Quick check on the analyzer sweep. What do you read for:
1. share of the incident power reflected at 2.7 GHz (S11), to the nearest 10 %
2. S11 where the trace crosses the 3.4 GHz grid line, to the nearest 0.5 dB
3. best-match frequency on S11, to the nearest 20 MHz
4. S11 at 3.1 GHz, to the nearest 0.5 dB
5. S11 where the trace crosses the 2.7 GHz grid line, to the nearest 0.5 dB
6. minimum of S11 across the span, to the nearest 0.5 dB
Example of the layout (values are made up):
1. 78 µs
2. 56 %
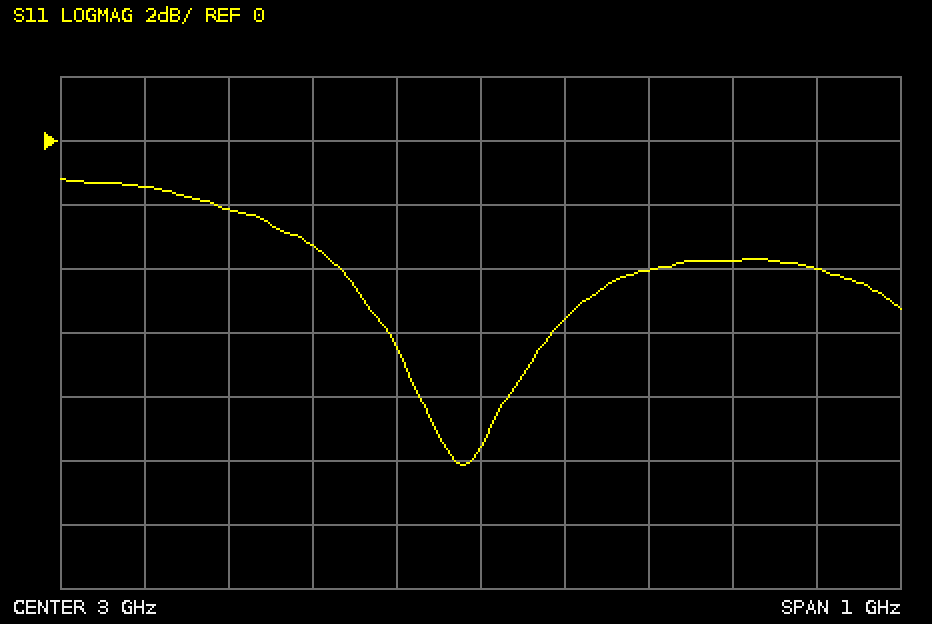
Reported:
1. 60 %
2. -4.0 dB
3. 2.98 GHz
4. -5.5 dB
5. -2.0 dB
6. -10.0 dB
